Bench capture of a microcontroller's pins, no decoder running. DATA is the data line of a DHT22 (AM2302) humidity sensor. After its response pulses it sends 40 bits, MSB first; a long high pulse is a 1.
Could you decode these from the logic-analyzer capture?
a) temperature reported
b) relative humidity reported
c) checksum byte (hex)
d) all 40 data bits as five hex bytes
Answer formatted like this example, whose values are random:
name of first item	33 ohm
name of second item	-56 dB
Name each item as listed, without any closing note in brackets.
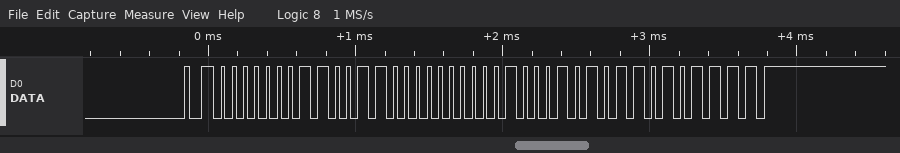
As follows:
temperature reported	27.7 °C
relative humidity reported	40.8 %
checksum byte	0xAF
all 40 data bits as five hex bytes	01 98 01 15 AF
